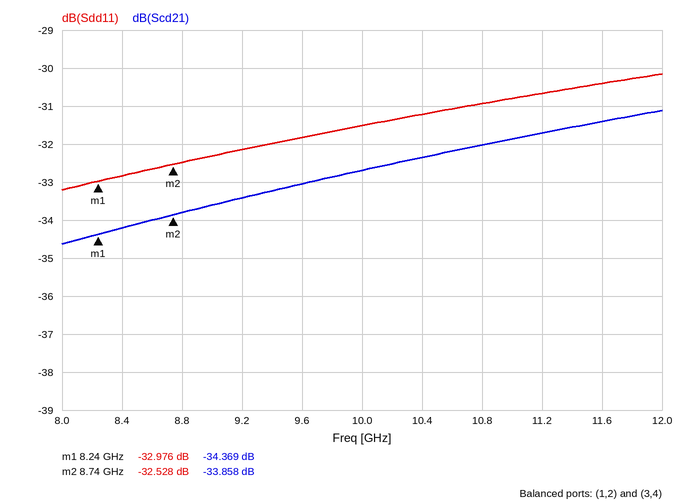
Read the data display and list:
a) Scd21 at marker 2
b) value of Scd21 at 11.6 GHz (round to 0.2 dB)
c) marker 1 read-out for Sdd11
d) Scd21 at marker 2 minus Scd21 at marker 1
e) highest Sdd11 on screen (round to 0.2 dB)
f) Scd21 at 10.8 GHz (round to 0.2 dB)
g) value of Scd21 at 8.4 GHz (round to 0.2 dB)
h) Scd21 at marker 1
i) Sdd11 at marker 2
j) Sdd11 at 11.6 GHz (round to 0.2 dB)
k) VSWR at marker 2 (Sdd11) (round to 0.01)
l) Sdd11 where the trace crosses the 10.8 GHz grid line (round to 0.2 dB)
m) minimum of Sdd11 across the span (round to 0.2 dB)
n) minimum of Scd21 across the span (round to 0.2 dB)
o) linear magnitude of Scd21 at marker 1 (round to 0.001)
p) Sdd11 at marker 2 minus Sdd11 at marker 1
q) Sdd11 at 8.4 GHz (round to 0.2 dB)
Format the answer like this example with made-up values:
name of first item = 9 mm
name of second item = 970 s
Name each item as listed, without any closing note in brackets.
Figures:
Scd21 at marker 2 = -33.858 dB
value of Scd21 at 11.6 GHz = -31.4 dB
marker 1 read-out for Sdd11 = -32.976 dB
Scd21 at marker 2 minus Scd21 at marker 1 = 0.511 dB
highest Sdd11 on screen = -30.2 dB
Scd21 at 10.8 GHz = -32.0 dB
value of Scd21 at 8.4 GHz = -34.2 dB
Scd21 at marker 1 = -34.369 dB
Sdd11 at marker 2 = -32.528 dB
Sdd11 at 11.6 GHz = -30.4 dB
VSWR at marker 2 (Sdd11) = 1.05
Sdd11 where the trace crosses the 10.8 GHz grid line = -31.0 dB
minimum of Sdd11 across the span = -33.2 dB
minimum of Scd21 across the span = -34.6 dB
linear magnitude of Scd21 at marker 1 = 0.019
Sdd11 at marker 2 minus Sdd11 at marker 1 = 0.448 dB
Sdd11 at 8.4 GHz = -32.8 dB
